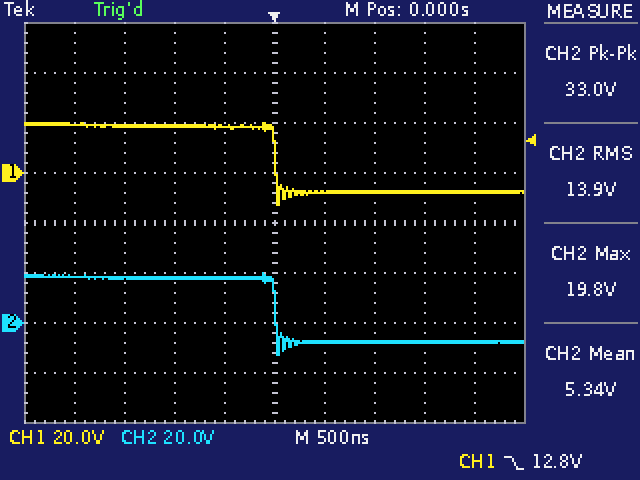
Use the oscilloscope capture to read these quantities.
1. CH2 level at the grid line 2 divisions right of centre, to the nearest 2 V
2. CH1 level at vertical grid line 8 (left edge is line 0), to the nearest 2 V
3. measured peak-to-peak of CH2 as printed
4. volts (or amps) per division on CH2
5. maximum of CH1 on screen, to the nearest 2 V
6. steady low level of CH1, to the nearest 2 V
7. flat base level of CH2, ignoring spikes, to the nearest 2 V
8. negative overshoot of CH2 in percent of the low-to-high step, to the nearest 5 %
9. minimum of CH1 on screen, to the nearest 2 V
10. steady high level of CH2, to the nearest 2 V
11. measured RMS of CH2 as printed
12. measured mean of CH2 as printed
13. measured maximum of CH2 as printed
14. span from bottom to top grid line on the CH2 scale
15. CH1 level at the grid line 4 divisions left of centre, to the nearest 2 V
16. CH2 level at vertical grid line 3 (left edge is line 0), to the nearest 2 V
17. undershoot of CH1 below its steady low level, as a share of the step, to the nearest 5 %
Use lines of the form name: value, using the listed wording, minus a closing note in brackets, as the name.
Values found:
CH2 level at the grid line 2 divisions right of centre, to the nearest 2 V: -8 V
CH1 level at vertical grid line 8 (left edge is line 0), to the nearest 2 V: -8 V
measured peak-to-peak of CH2 as printed: 33.0 V
volts (or amps) per division on CH2: 20 V
maximum of CH1 on screen, to the nearest 2 V: 20 V
steady low level of CH1, to the nearest 2 V: -8 V
flat base level of CH2, ignoring spikes, to the nearest 2 V: -8 V
negative overshoot of CH2 in percent of the low-to-high step, to the nearest 5 %: 20 %
minimum of CH1 on screen, to the nearest 2 V: -12 V
steady high level of CH2, to the nearest 2 V: 18 V
measured RMS of CH2 as printed: 13.9 V
measured mean of CH2 as printed: 5.34 V
measured maximum of CH2 as printed: 19.8 V
span from bottom to top grid line on the CH2 scale: 160 V
CH1 level at the grid line 4 divisions left of centre, to the nearest 2 V: 20 V
CH2 level at vertical grid line 3 (left edge is line 0), to the nearest 2 V: 18 V
undershoot of CH1 below its steady low level, as a share of the step, to the nearest 5 %: 20 %
